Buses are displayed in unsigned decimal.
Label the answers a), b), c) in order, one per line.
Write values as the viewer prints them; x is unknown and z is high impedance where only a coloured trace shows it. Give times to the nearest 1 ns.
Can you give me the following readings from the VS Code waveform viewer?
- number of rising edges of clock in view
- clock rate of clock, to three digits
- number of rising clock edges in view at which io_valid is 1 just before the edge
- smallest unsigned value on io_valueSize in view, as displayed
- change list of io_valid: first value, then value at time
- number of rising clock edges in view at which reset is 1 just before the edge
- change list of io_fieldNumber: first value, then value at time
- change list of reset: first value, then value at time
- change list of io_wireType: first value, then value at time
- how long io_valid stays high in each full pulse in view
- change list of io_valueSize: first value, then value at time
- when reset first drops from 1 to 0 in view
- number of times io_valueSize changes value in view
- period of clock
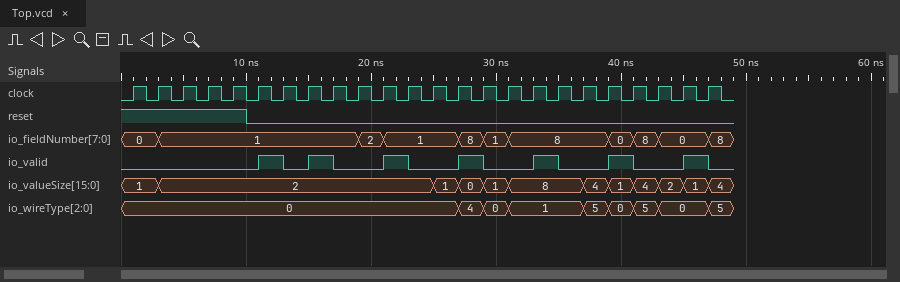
a) 24
b) 500 MHz
c) 7
d) 0
e) 0, 1 at 11 ns, 0 at 13 ns, 1 at 15 ns, 0 at 17 ns, 1 at 21 ns, 0 at 23 ns, 1 at 27 ns, 0 at 29 ns, 1 at 33 ns, 0 at 35 ns, 1 at 39 ns, 0 at 41 ns, 1 at 45 ns, 0 at 47 ns
f) 5
g) 0, 1 at 3 ns, 2 at 19 ns, 1 at 21 ns, 8 at 27 ns, 1 at 29 ns, 8 at 31 ns, 0 at 39 ns, 8 at 41 ns, 0 at 43 ns, 8 at 47 ns
h) 1, 0 at 10 ns
i) 0, 4 at 27 ns, 0 at 29 ns, 1 at 31 ns, 5 at 37 ns, 0 at 39 ns, 5 at 41 ns, 0 at 43 ns, 5 at 47 ns
j) 2 ns, 2 ns, 2 ns, 2 ns, 2 ns, 2 ns, 2 ns
k) 1, 2 at 3 ns, 1 at 25 ns, 0 at 27 ns, 1 at 29 ns, 8 at 31 ns, 4 at 37 ns, 1 at 39 ns, 4 at 41 ns, 2 at 43 ns, 1 at 45 ns, 4 at 47 ns
l) 10 ns
m) 11
n) 2 ns
